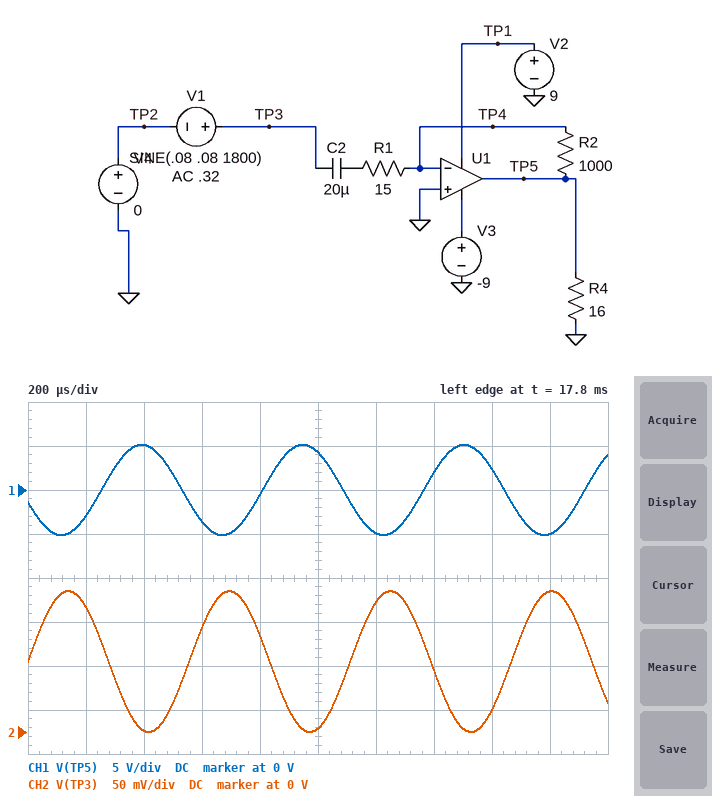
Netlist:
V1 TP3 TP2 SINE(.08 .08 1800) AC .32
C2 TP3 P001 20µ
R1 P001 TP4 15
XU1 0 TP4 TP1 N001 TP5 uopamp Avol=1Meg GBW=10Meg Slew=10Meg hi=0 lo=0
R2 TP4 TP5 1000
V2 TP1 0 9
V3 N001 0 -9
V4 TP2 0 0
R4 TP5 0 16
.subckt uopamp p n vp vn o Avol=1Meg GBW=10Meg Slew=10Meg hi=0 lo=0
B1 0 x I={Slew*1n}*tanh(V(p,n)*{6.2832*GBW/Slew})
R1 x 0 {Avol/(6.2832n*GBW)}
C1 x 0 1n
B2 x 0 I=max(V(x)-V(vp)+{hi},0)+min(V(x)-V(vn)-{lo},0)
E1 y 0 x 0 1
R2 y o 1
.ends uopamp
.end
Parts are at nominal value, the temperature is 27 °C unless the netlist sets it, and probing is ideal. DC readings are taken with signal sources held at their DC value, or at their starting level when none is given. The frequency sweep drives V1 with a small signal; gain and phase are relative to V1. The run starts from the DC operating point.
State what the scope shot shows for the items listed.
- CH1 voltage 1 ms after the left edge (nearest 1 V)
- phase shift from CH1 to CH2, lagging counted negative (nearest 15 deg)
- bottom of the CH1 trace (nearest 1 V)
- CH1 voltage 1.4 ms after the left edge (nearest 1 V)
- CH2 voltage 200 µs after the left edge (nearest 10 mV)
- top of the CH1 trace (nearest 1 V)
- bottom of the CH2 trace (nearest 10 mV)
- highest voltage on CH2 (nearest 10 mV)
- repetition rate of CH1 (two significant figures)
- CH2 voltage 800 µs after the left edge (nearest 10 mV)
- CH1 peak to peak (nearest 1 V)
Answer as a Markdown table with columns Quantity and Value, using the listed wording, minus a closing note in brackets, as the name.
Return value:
| Quantity | Value |
|---|---|
| CH1 voltage 1 ms after the left edge | 4 V |
| phase shift from CH1 to CH2, lagging counted negative | 165 deg |
| bottom of the CH1 trace | -5 V |
| CH1 voltage 1.4 ms after the left edge | 2 V |
| CH2 voltage 200 µs after the left edge | 140 mV |
| top of the CH1 trace | 5 V |
| bottom of the CH2 trace | 0 V |
| highest voltage on CH2 | 160 mV |
| repetition rate of CH1 | 1.8 kHz |
| CH2 voltage 800 µs after the left edge | 110 mV |
| CH1 peak to peak | 10 V |
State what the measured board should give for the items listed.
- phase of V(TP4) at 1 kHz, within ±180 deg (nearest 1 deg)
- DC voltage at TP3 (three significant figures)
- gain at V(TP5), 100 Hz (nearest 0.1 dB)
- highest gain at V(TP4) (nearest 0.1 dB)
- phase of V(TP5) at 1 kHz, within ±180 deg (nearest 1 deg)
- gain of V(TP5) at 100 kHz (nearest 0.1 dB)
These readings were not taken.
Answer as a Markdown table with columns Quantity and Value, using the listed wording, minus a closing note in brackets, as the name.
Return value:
| Quantity | Value |
|---|---|
| phase of V(TP4) at 1 kHz, within ±180 deg | 117 deg |
| DC voltage at TP3 | 80.0 mV |
| gain at V(TP5), 100 Hz | 21.8 dB |
| highest gain at V(TP4) | -0.1 dB |
| phase of V(TP5) at 1 kHz, within ±180 deg | -152 deg |
| gain of V(TP5) at 100 kHz | 34.7 dB |
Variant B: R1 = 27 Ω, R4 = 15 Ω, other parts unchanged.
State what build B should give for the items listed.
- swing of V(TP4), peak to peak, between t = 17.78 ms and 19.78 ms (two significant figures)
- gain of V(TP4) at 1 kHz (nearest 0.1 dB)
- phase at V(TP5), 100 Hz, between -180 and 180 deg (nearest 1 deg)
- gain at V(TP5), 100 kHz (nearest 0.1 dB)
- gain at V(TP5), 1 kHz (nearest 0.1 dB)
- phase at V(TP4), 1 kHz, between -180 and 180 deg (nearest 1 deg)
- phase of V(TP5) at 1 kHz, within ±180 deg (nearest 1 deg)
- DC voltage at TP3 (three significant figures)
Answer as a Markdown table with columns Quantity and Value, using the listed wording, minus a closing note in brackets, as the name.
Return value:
| Quantity | Value |
|---|---|
| swing of V(TP4), peak to peak, between t = 17.78 ms and 19.78 ms | 1.1 mV |
| gain of V(TP4) at 1 kHz | -48.4 dB |
| phase at V(TP5), 100 Hz, between -180 and 180 deg | -109 deg |
| gain at V(TP5), 100 kHz | 30.7 dB |
| gain at V(TP5), 1 kHz | 31.0 dB |
| phase at V(TP4), 1 kHz, between -180 and 180 deg | 106 deg |
| phase of V(TP5) at 1 kHz, within ±180 deg | -164 deg |
| DC voltage at TP3 | 80.0 mV |
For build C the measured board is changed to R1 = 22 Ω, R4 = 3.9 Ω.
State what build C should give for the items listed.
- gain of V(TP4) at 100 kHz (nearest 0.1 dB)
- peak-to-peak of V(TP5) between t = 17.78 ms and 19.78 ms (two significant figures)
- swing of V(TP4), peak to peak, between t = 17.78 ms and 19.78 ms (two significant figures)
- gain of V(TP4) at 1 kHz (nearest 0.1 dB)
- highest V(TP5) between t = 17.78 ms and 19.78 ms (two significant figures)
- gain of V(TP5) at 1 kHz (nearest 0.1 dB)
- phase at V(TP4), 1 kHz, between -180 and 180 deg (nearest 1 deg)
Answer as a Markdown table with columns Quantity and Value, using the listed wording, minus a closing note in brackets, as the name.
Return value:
| Quantity | Value |
|---|---|
| gain of V(TP4) at 100 kHz | -6.1 dB |
| peak-to-peak of V(TP5) between t = 17.78 ms and 19.78 ms | 7.1 V |
| swing of V(TP4), peak to peak, between t = 17.78 ms and 19.78 ms | 1.6 mV |
| gain of V(TP4) at 1 kHz | -45.4 dB |
| highest V(TP5) between t = 17.78 ms and 19.78 ms | 3.6 V |
| gain of V(TP5) at 1 kHz | 32.6 dB |
| phase at V(TP4), 1 kHz, between -180 and 180 deg | 109 deg |
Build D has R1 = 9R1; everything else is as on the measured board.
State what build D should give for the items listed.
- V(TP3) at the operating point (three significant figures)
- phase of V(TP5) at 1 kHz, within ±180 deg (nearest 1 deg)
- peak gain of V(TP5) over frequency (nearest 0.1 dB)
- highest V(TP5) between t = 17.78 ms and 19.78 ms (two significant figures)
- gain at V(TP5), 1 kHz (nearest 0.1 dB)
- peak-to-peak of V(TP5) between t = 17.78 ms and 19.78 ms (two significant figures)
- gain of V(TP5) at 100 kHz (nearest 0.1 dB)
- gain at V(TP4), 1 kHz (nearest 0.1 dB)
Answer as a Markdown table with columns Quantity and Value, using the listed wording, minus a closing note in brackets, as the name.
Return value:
| Quantity | Value |
|---|---|
| V(TP3) at the operating point | 80.0 mV |
| phase of V(TP5) at 1 kHz, within ±180 deg | -139 deg |
| peak gain of V(TP5) over frequency | 40.8 dB |
| highest V(TP5) between t = 17.78 ms and 19.78 ms | 8.0 V |
| gain at V(TP5), 1 kHz | 38.4 dB |
| peak-to-peak of V(TP5) between t = 17.78 ms and 19.78 ms | 16 V |
| gain of V(TP5) at 100 kHz | 37.1 dB |
| gain at V(TP4), 1 kHz | -41.1 dB |
